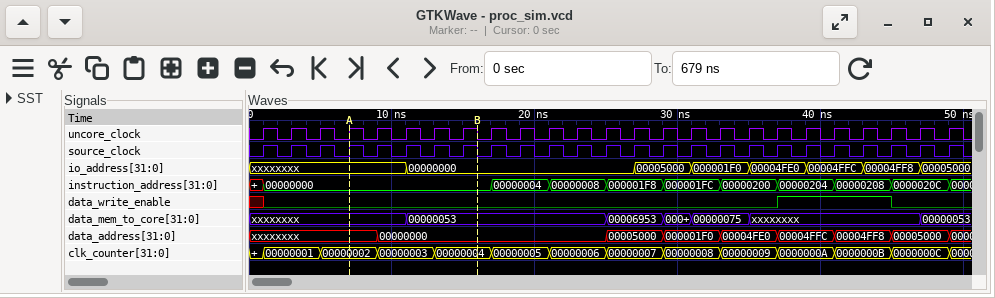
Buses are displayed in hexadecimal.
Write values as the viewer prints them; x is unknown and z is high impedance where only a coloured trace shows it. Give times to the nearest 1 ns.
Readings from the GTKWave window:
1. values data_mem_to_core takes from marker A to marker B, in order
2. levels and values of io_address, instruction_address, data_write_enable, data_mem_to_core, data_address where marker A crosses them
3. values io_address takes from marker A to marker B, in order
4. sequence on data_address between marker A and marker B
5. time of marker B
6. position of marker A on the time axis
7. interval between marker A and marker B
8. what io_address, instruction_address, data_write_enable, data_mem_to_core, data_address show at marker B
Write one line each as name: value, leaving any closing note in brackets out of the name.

values data_mem_to_core takes from marker A to marker B, in order: xxxxxxxx, 00000053
levels and values of io_address, instruction_address, data_write_enable, data_mem_to_core, data_address where marker A crosses them: io_address=xxxxxxxx, instruction_address=00000000, data_write_enable=0, data_mem_to_core=xxxxxxxx, data_address=xxxxxxxx
values io_address takes from marker A to marker B, in order: xxxxxxxx, 00000000
sequence on data_address between marker A and marker B: xxxxxxxx, 00000000
time of marker B: 16 ns
position of marker A on the time axis: 7 ns
interval between marker A and marker B: 9 ns
what io_address, instruction_address, data_write_enable, data_mem_to_core, data_address show at marker B: io_address=00000000, instruction_address=00000000, data_write_enable=0, data_mem_to_core=00000053, data_address=00000000
